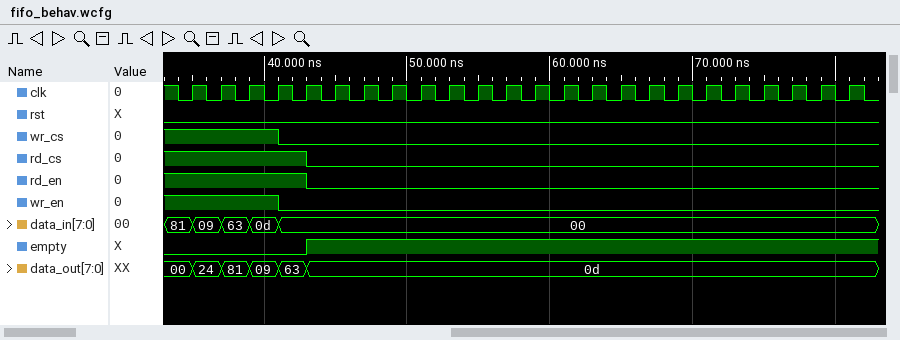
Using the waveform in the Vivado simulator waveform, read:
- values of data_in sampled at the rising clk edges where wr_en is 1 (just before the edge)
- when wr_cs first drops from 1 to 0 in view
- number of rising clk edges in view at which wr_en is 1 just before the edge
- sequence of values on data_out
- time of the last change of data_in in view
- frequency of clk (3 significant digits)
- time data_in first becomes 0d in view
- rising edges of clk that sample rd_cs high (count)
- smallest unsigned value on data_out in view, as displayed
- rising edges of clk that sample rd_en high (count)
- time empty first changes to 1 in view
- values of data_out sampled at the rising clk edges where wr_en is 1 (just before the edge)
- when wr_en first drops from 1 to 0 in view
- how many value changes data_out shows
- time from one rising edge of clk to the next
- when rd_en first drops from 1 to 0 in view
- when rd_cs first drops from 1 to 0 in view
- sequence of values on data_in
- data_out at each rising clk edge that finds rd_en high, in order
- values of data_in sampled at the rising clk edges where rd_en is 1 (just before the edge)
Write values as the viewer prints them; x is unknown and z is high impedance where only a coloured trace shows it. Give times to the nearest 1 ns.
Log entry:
81, 09, 63, 0d
41 ns
4
00, 24, 81, 09, 63, 0d
41 ns
500 MHz
39 ns
5
00
5
43 ns
00, 24, 81, 09
41 ns
5
2 ns
43 ns
43 ns
81, 09, 63, 0d, 00
00, 24, 81, 09, 63
81, 09, 63, 0d, 00
